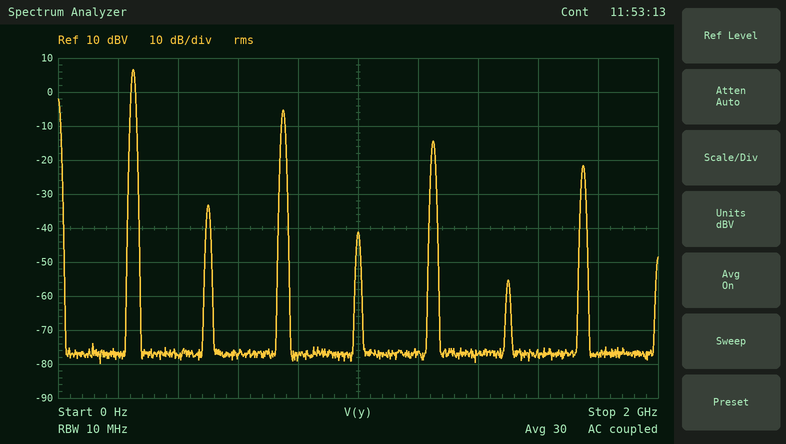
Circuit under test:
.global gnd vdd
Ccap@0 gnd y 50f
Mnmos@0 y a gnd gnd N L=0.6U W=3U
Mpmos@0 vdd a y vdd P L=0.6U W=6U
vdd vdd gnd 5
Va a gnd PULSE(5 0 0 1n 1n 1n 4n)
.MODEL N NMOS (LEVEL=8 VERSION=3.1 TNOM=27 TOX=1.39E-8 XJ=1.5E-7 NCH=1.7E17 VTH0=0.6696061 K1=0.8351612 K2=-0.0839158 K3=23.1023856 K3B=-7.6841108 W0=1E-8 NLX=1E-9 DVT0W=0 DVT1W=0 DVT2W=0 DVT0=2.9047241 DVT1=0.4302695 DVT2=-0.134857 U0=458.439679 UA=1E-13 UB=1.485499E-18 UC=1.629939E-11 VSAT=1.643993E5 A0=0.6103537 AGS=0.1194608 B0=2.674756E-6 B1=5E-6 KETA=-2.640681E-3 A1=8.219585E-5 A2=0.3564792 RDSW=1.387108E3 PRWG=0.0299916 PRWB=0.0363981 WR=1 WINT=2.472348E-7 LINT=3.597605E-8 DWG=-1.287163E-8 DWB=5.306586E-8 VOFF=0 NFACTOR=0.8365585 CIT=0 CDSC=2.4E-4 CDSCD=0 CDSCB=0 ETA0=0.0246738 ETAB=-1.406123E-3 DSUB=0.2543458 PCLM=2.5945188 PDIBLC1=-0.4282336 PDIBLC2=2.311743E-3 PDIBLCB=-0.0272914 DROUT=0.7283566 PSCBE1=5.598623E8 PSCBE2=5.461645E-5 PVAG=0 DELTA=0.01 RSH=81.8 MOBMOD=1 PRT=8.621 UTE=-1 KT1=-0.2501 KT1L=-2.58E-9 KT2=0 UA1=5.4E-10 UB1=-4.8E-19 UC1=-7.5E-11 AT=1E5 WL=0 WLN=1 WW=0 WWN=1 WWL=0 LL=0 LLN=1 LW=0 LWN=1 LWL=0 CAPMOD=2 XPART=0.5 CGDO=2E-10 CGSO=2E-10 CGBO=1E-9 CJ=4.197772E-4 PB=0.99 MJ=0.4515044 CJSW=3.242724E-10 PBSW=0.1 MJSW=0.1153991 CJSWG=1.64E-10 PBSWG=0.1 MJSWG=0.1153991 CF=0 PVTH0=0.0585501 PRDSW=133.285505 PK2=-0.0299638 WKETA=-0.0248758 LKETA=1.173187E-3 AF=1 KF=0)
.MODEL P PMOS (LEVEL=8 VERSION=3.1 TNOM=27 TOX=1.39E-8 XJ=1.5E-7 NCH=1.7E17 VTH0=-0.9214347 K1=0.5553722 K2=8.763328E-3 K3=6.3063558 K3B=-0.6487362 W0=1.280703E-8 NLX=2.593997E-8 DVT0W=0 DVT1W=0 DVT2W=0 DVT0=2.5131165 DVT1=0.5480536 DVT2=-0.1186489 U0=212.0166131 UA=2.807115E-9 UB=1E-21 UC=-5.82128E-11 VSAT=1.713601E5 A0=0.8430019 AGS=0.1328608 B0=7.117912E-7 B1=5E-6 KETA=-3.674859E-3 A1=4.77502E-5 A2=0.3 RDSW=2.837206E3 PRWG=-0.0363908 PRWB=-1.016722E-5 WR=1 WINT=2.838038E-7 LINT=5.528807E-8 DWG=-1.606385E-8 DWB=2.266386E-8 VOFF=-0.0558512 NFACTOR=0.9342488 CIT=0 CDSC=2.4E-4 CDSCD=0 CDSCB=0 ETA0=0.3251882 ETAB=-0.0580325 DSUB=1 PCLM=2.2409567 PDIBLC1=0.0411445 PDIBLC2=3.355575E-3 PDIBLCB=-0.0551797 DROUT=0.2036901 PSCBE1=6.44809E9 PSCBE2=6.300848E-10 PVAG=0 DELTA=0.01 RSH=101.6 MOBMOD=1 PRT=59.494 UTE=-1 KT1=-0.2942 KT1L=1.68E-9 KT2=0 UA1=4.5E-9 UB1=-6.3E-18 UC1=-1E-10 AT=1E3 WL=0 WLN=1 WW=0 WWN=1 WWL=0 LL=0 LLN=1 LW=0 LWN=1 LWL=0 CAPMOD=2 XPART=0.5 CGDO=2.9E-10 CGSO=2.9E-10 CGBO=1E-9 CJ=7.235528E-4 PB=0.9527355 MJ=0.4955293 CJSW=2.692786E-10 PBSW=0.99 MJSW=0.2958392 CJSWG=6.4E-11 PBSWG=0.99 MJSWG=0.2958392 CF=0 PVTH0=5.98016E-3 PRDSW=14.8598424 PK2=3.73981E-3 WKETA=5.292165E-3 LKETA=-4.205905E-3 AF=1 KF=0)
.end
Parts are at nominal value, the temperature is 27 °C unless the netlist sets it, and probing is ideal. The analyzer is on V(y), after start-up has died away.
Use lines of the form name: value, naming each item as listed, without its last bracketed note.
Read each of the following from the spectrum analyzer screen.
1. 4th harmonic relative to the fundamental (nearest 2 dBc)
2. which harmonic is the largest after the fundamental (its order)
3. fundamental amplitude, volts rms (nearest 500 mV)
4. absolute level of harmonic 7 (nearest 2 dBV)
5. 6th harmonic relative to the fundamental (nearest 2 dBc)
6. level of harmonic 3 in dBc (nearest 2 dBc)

4th harmonic relative to the fundamental: -48 dBc
which harmonic is the largest after the fundamental: 3
fundamental amplitude, volts rms: 2.0 V
absolute level of harmonic 7: -22 dBV
6th harmonic relative to the fundamental: -62 dBc
level of harmonic 3 in dBc: -12 dBc
